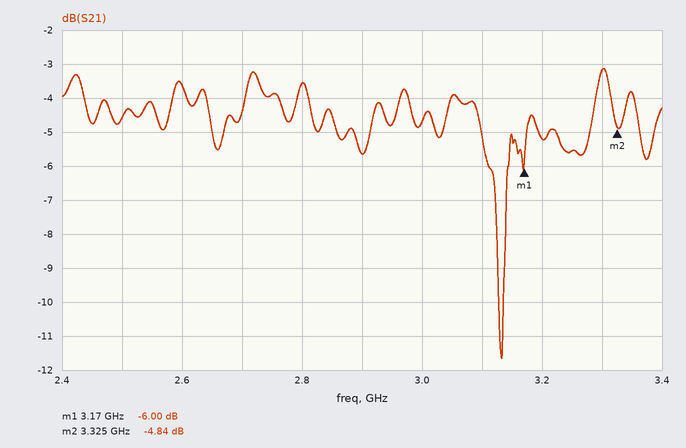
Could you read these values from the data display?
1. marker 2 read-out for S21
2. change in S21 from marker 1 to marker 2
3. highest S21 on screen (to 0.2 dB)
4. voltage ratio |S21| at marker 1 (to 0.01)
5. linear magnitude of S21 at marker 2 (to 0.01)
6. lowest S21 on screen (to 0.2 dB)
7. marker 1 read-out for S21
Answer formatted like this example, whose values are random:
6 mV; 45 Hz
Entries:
-4.84 dB; 1.16 dB; -3.2 dB; 0.50; 0.57; -11.6 dB; -6.00 dB
